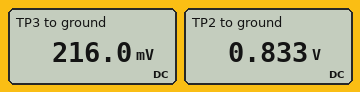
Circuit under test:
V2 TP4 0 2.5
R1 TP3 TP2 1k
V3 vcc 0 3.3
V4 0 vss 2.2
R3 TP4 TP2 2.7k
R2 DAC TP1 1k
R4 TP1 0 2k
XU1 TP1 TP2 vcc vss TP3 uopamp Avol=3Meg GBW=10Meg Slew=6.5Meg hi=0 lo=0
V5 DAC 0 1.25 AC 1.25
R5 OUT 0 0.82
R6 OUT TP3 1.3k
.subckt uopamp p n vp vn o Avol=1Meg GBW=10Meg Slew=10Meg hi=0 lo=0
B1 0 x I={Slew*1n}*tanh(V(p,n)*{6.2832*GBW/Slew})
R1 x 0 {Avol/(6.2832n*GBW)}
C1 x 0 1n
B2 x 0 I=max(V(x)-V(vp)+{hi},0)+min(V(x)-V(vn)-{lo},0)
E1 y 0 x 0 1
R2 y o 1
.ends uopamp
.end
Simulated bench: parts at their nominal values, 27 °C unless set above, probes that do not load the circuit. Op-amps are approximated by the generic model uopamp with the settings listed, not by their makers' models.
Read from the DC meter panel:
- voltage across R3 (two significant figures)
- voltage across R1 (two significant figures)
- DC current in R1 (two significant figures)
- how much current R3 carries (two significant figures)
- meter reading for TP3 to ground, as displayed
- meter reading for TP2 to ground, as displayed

1.7 V
620 mV
620 µA
620 µA
216.0 mV
0.833 V
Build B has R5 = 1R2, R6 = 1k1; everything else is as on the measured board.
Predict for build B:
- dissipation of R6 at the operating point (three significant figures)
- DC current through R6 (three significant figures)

42.3 µW
196 µA
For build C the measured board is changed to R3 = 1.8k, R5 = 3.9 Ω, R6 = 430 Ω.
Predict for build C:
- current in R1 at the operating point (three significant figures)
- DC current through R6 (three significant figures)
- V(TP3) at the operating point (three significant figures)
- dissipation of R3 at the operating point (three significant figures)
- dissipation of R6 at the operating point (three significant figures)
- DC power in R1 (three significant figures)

926 µA
213 µA
-92.6 mV
1.54 mW
19.6 µW
857 µW
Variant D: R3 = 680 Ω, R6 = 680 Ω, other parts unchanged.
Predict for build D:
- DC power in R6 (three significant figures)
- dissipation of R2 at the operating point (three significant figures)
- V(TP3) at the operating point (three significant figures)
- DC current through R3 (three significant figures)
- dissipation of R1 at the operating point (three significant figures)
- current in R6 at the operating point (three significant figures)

3.84 mW
174 µW
-1.62 V
2.45 mA
6.01 mW
2.38 mA
